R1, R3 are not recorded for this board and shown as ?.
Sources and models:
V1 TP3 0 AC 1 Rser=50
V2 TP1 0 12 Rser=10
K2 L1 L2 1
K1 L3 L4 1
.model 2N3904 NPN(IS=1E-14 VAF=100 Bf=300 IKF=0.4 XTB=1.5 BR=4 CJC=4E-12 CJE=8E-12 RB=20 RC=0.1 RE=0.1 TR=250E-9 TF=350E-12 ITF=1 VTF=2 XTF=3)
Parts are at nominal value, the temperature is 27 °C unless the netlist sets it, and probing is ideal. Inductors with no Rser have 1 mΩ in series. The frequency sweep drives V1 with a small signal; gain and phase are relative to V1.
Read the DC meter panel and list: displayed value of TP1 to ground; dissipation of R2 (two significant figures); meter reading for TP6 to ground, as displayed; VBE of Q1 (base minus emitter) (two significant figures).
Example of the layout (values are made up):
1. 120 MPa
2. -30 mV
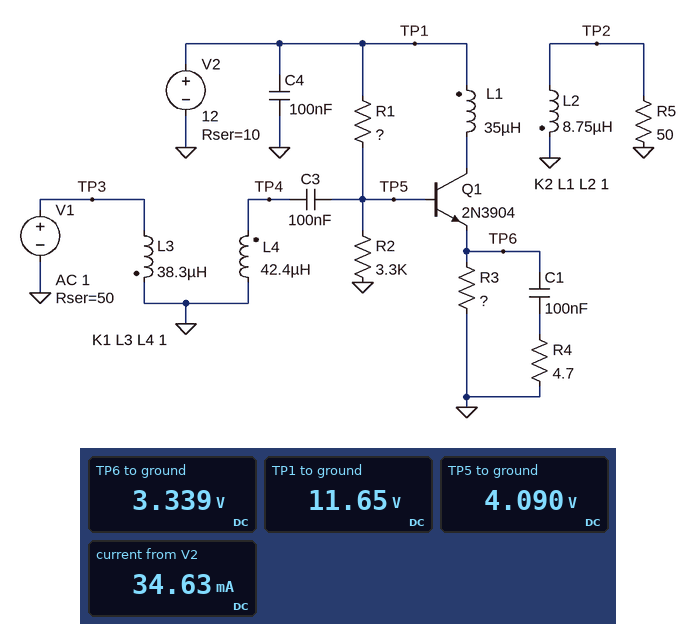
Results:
1. 11.65 V
2. 5.1 mW
3. 3.339 V
4. 750 mV
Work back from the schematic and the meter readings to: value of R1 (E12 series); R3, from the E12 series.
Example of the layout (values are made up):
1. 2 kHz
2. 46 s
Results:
1. 5.6 kΩ
2. 100 Ω
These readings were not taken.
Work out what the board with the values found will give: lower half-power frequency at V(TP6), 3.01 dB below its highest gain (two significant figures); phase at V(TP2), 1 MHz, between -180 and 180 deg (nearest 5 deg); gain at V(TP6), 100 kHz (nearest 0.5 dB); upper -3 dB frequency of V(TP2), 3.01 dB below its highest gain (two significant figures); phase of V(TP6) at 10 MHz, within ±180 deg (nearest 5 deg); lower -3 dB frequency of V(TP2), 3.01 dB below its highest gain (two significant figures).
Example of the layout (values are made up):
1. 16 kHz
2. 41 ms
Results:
1. 150 kHz
2. 65 deg
3. -7.0 dB
4. 17 MHz
5. 150 deg
6. 940 kHz
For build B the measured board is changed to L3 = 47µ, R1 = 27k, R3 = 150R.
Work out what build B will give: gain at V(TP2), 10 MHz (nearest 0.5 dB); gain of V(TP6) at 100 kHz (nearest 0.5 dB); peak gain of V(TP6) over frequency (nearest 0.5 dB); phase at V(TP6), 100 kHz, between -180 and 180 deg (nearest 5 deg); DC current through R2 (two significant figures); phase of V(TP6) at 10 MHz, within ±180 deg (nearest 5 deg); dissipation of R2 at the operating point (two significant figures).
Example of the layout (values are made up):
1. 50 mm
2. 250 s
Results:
1. 18.0 dB
2. -8.0 dB
3. -7.0 dB
4. -140 deg
5. 380 µA
6. 165 deg
7. 490 µW
